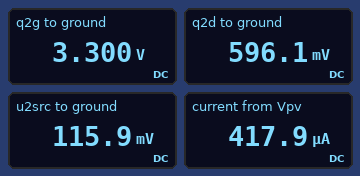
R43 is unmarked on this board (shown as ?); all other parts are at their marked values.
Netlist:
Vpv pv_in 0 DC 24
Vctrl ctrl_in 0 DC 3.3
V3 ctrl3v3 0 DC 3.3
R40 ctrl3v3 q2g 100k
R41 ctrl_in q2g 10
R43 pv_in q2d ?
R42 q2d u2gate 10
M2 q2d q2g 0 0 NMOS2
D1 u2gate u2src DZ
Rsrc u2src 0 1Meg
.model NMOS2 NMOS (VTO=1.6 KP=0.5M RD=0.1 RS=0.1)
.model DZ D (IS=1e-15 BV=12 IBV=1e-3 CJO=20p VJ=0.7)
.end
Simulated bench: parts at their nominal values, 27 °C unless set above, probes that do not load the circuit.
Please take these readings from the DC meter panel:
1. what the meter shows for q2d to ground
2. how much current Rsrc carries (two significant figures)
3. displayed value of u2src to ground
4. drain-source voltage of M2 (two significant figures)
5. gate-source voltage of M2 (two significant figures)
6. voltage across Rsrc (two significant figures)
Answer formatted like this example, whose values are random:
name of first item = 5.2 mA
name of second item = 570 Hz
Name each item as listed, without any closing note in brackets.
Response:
what the meter shows for q2d to ground = 596.1 mV
how much current Rsrc carries = 120 nA
displayed value of u2src to ground = 115.9 mV
drain-source voltage of M2 = 600 mV
gate-source voltage of M2 = 3.3 V
voltage across Rsrc = 120 mV
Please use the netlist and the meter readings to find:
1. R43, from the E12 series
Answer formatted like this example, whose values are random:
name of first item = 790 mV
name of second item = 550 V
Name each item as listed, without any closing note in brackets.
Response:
R43, from the E12 series = 56 kΩ
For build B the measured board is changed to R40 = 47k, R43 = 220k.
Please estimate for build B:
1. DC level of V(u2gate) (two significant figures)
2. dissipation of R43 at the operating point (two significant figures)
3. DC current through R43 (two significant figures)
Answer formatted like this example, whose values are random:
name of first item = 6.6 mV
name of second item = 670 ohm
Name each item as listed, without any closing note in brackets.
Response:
DC level of V(u2gate) = 130 mV
dissipation of R43 at the operating point = 2.6 mW
DC current through R43 = 110 µA
